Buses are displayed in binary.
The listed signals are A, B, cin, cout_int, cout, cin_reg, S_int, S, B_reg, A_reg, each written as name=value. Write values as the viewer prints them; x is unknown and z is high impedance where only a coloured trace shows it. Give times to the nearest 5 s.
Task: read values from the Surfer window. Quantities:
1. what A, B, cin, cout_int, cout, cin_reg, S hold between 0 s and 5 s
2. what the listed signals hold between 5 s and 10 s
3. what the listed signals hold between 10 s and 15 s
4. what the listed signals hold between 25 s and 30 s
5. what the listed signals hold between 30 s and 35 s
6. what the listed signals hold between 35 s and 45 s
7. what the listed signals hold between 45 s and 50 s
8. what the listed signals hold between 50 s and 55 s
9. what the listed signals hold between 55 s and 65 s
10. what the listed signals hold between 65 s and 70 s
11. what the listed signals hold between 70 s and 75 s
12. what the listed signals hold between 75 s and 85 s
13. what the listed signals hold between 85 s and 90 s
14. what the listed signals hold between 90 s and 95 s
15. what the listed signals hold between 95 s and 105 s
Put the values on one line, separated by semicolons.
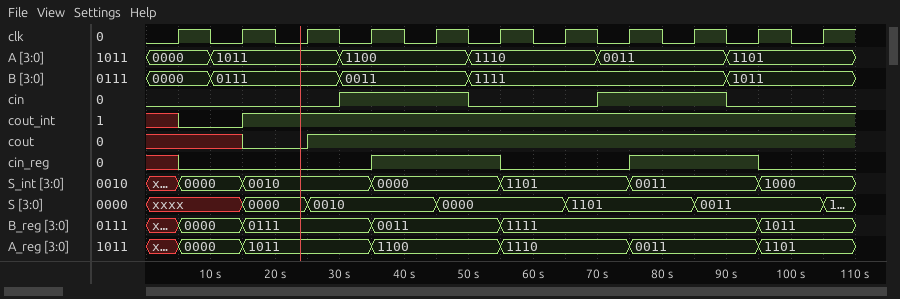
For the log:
A=0000, B=0000, cin=0, cout_int=x, cout=x, cin_reg=x, S=xxxx; A=0000, B=0000, cin=0, cout_int=0, cout=x, cin_reg=0, S_int=0000, S=xxxx, B_reg=0000, A_reg=0000; A=1011, B=0111, cin=0, cout_int=0, cout=x, cin_reg=0, S_int=0000, S=xxxx, B_reg=0000, A_reg=0000; A=1011, B=0111, cin=0, cout_int=1, cout=1, cin_reg=0, S_int=0010, S=0010, B_reg=0111, A_reg=1011; A=1100, B=0011, cin=1, cout_int=1, cout=1, cin_reg=0, S_int=0010, S=0010, B_reg=0111, A_reg=1011; A=1100, B=0011, cin=1, cout_int=1, cout=1, cin_reg=1, S_int=0000, S=0010, B_reg=0011, A_reg=1100; A=1100, B=0011, cin=1, cout_int=1, cout=1, cin_reg=1, S_int=0000, S=0000, B_reg=0011, A_reg=1100; A=1110, B=1111, cin=0, cout_int=1, cout=1, cin_reg=1, S_int=0000, S=0000, B_reg=0011, A_reg=1100; A=1110, B=1111, cin=0, cout_int=1, cout=1, cin_reg=0, S_int=1101, S=0000, B_reg=1111, A_reg=1110; A=1110, B=1111, cin=0, cout_int=1, cout=1, cin_reg=0, S_int=1101, S=1101, B_reg=1111, A_reg=1110; A=0011, B=1111, cin=1, cout_int=1, cout=1, cin_reg=0, S_int=1101, S=1101, B_reg=1111, A_reg=1110; A=0011, B=1111, cin=1, cout_int=1, cout=1, cin_reg=1, S_int=0011, S=1101, B_reg=1111, A_reg=0011; A=0011, B=1111, cin=1, cout_int=1, cout=1, cin_reg=1, S_int=0011, S=0011, B_reg=1111, A_reg=0011; A=1101, B=1011, cin=0, cout_int=1, cout=1, cin_reg=1, S_int=0011, S=0011, B_reg=1111, A_reg=0011; A=1101, B=1011, cin=0, cout_int=1, cout=1, cin_reg=0, S_int=1000, S=0011, B_reg=1011, A_reg=1101
